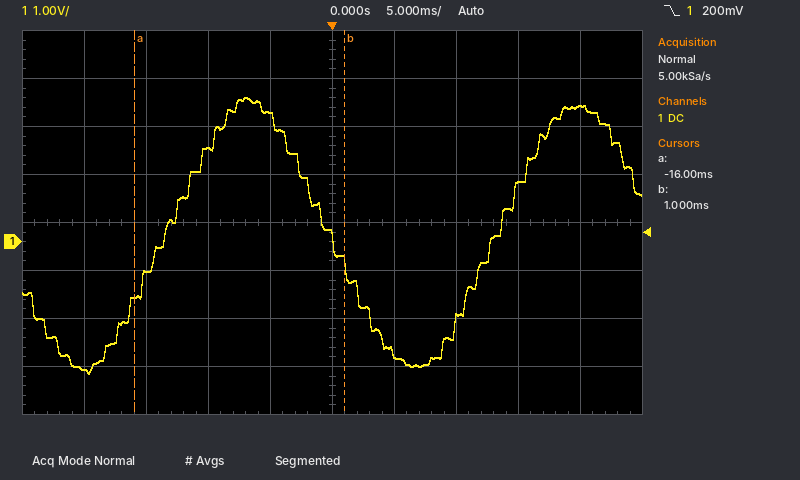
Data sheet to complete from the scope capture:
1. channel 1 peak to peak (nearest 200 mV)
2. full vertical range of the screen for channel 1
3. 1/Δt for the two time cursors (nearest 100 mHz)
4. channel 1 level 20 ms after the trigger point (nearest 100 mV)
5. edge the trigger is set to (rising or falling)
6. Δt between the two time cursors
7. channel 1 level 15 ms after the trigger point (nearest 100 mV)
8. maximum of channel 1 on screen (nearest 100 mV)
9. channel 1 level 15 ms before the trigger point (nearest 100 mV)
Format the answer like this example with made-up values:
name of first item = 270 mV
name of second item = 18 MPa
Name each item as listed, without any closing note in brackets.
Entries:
channel 1 peak to peak = 5.8 V
full vertical range of the screen for channel 1 = 8 V
1/Δt for the two time cursors = 58.8 Hz
channel 1 level 20 ms after the trigger point = 2.8 V
edge the trigger is set to = falling
Δt between the two time cursors = 17.0 ms
channel 1 level 15 ms after the trigger point = 1.2 V
maximum of channel 1 on screen = 3.0 V
channel 1 level 15 ms before the trigger point = -600 mV
